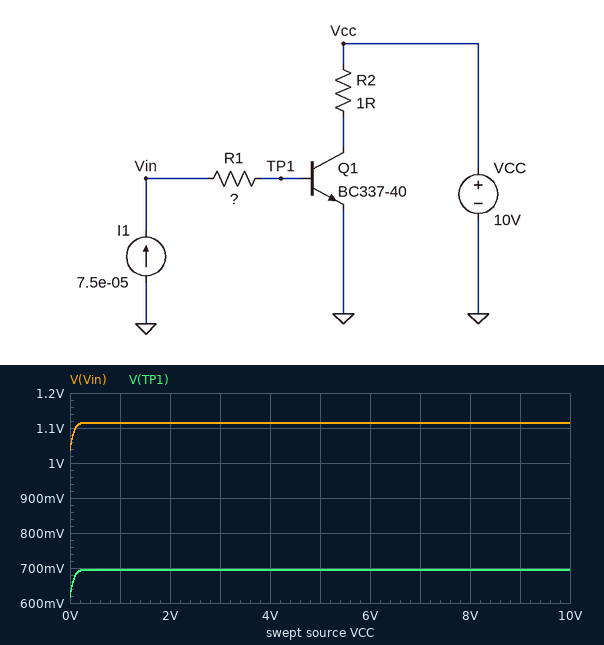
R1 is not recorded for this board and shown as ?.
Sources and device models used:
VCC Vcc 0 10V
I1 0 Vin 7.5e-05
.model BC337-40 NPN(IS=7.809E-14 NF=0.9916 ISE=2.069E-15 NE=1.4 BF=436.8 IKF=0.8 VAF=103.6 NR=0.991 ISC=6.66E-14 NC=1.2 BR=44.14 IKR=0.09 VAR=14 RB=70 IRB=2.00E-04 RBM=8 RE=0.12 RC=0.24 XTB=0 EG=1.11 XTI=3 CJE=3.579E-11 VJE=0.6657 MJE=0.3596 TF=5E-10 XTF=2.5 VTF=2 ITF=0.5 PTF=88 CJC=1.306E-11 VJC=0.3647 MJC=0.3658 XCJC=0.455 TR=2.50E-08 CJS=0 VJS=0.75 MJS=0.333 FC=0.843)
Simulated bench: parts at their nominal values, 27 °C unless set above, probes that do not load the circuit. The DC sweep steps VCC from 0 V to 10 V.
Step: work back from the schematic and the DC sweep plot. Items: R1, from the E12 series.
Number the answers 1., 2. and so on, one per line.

1. 5.6 kΩ
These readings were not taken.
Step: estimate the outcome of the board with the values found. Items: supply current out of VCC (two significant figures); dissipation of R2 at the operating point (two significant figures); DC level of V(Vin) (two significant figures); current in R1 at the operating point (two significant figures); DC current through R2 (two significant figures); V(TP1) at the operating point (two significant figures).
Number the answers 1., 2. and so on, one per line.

1. 33 mA
2. 1.1 mW
3. 1.1 V
4. 75 µA
5. 33 mA
6. 690 mV
